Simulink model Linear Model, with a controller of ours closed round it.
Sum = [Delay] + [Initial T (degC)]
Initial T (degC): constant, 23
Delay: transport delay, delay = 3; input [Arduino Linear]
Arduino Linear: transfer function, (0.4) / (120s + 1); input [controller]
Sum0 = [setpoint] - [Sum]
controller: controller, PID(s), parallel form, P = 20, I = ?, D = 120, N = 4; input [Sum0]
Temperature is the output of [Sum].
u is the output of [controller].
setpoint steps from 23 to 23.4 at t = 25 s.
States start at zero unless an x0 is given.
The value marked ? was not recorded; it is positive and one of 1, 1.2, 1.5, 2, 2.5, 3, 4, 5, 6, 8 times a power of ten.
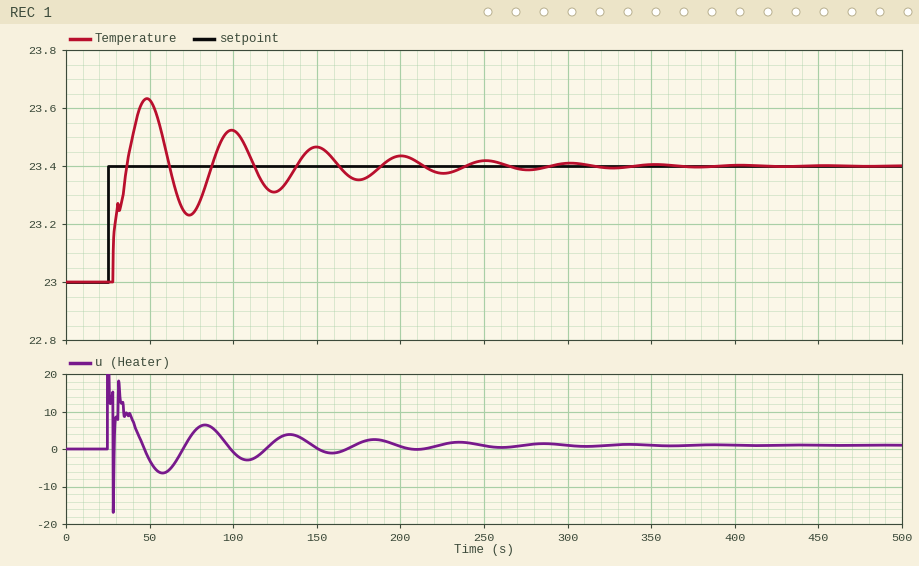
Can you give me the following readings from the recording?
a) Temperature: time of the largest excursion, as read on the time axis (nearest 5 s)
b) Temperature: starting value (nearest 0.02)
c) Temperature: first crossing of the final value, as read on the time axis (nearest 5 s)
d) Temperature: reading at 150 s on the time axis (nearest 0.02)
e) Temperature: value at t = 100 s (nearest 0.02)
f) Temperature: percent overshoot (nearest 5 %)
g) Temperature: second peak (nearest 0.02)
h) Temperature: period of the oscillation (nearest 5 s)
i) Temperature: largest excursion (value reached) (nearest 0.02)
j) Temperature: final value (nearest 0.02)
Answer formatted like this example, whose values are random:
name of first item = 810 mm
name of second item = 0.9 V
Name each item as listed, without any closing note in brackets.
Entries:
Temperature: time of the largest excursion, as read on the time axis = 50 s
Temperature: starting value = 23.00
Temperature: first crossing of the final value, as read on the time axis = 35 s
Temperature: reading at 150 s on the time axis = 23.46
Temperature: value at t = 100 s = 23.52
Temperature: percent overshoot = 60 %
Temperature: second peak = 23.52
Temperature: period of the oscillation = 50 s
Temperature: largest excursion (value reached) = 23.64
Temperature: final value = 23.40
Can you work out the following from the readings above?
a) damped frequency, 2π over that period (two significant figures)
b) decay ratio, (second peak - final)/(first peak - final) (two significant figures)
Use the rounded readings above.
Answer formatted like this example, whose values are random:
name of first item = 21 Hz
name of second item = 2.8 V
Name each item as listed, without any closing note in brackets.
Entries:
damped frequency, 2π over that period = 0.13 rad/s
decay ratio, (second peak - final)/(first peak - final) = 0.50
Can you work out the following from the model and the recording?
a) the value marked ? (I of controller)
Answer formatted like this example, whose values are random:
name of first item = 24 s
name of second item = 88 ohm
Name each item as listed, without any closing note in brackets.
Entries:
the value marked ? = 6
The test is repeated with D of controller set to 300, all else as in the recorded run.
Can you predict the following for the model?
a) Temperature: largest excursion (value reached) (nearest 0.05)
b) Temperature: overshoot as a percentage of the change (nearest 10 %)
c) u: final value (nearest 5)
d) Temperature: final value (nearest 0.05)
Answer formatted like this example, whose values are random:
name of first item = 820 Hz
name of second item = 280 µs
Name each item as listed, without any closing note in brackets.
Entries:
Temperature: largest excursion (value reached) = 23.75
Temperature: overshoot as a percentage of the change = 90 %
u: final value = 0
Temperature: final value = 23.40
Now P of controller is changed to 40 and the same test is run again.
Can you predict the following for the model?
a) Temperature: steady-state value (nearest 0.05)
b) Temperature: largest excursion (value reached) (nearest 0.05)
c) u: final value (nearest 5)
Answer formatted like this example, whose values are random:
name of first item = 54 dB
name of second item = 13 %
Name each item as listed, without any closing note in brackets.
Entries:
Temperature: steady-state value = 23.40
Temperature: largest excursion (value reached) = 23.55
u: final value = 0
